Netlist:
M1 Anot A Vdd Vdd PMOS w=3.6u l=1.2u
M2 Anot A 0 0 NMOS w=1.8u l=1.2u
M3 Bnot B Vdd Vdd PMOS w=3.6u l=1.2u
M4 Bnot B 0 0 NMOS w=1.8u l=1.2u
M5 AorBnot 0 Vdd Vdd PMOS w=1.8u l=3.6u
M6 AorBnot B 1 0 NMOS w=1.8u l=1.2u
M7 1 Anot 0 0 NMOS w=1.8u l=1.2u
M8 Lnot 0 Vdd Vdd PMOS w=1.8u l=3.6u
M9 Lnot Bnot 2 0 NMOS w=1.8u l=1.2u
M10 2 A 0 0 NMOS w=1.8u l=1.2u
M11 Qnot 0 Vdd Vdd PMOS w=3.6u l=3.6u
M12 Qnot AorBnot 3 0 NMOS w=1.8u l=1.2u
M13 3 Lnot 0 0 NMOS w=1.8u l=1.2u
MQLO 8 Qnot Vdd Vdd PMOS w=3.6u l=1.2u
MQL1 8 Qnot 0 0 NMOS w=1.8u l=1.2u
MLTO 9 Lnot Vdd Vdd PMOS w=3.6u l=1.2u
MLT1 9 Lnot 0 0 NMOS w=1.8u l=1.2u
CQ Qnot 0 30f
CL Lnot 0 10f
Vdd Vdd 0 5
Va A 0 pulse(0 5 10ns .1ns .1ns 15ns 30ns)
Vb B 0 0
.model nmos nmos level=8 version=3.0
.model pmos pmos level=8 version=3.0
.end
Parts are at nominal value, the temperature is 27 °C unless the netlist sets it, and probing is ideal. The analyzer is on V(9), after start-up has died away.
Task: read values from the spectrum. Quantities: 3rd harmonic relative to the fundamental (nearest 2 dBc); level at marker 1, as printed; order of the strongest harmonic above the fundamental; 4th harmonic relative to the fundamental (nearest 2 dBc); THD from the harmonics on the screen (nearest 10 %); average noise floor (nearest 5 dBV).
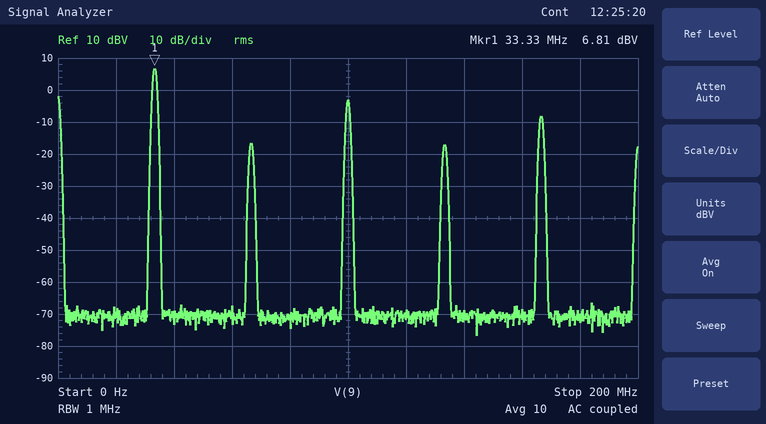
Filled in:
-10 dBc
6.81 dBV
3
-24 dBc
40 %
-70 dBV
